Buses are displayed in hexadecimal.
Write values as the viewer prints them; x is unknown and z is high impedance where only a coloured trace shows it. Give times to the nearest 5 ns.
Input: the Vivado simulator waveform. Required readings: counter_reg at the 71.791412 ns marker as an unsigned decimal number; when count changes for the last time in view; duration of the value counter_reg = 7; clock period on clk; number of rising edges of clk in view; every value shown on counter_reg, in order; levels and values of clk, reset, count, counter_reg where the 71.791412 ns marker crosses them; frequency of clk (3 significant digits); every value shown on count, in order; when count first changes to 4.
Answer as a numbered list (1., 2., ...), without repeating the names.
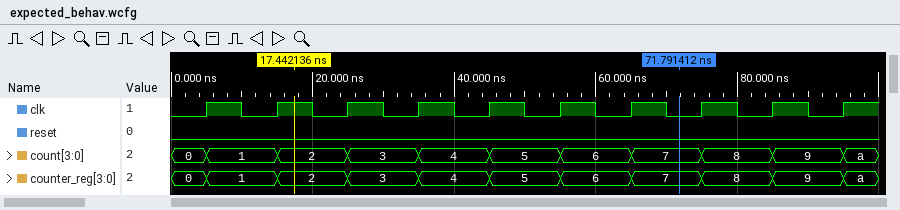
1. 7
2. 95 ns
3. 10 ns
4. 10 ns
5. 10
6. 0, 1, 2, 3, 4, 5, 6, 7, 8, 9, a
7. clk=0, reset=0, count=7, counter_reg=7
8. 100 MHz
9. 0, 1, 2, 3, 4, 5, 6, 7, 8, 9, a
10. 35 ns
